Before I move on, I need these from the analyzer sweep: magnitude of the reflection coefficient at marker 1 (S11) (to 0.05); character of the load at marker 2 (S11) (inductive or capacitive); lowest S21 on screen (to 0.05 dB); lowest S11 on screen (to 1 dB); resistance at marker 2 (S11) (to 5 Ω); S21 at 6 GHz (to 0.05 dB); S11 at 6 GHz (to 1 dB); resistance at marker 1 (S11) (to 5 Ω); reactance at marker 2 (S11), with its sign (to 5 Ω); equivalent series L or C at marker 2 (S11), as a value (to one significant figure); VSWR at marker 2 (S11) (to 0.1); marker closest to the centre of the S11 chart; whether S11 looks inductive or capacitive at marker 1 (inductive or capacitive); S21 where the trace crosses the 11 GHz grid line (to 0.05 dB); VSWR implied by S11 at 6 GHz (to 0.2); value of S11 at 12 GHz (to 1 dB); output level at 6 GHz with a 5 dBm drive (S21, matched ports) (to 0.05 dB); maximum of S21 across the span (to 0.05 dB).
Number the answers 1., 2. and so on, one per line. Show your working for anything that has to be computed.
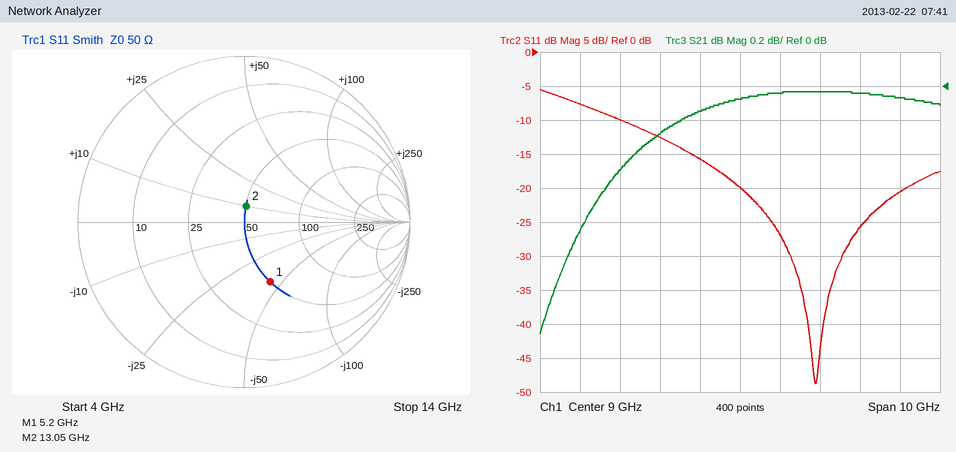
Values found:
1. 0.40
2. inductive
3. -1.45 dB
4. -49 dB
5. 50 Ω
6. -0.50 dB
7. -10 dB
8. 50 Ω
9. +10 Ω
10. L = 10 Ω/(2π × 13.05 GHz) ≈ 122 pH, so 100 pH to one significant figure
11. 1.2
12. marker 2
13. capacitive
14. -0.05 dB
15. |Γ| = 10^(-10/20) = 0.3162; VSWR = (1 + 0.3162)/(1 − 0.3162) ≈ 1.92, so 2.0 to the nearest 0.2
16. -26 dB
17. 5 dBm + (-0.50 dB) = 4.50 dBm
18. -0.05 dB
